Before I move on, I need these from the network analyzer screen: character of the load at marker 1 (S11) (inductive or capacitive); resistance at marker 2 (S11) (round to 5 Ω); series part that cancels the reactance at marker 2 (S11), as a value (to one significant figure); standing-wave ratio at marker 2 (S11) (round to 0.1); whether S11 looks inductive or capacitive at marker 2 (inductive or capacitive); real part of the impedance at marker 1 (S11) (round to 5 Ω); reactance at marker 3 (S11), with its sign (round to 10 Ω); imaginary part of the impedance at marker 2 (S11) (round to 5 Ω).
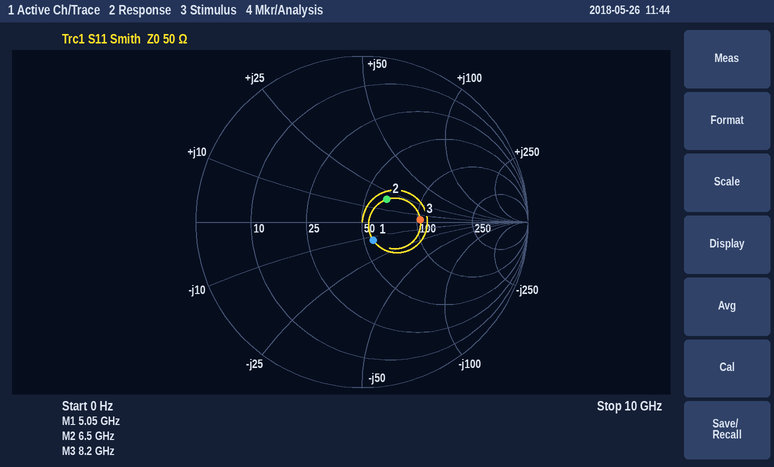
capacitive
65 Ω
1 pF
1.5
inductive
55 Ω
0 Ω
+20 Ω
